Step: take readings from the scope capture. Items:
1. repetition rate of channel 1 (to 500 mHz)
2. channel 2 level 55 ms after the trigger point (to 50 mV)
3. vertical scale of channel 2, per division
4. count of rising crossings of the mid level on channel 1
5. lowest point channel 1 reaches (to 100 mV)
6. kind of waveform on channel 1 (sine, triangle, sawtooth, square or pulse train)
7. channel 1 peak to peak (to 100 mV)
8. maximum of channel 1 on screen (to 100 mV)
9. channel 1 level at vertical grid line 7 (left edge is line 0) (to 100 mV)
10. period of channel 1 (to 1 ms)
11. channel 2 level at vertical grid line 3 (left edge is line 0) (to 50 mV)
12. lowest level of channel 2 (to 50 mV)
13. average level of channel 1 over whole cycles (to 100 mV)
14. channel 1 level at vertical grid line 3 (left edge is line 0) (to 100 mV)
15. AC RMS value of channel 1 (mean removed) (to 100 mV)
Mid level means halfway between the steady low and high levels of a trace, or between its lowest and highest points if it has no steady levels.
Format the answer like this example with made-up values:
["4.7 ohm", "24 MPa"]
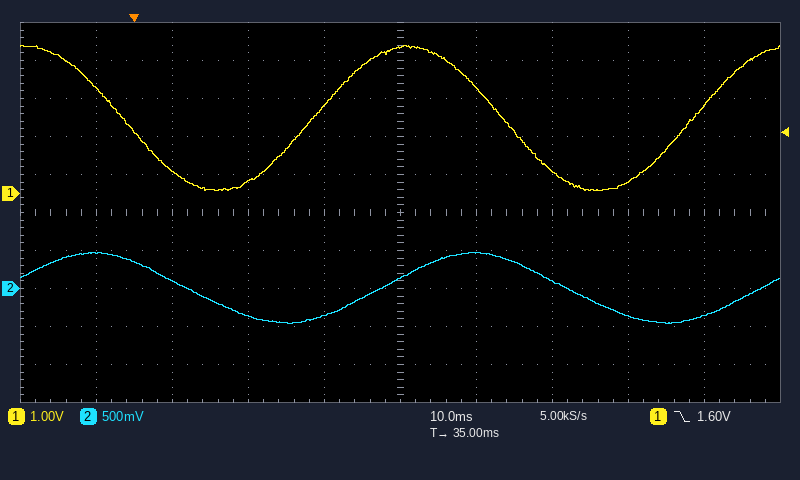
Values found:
["20.0 Hz", "100 mV", "500 mV", "2", "100 mV", "sine", "3.8 V", "3.9 V", "600 mV", "50 ms", "-350 mV", "-450 mV", "2.0 V", "300 mV", "1.3 V"]
